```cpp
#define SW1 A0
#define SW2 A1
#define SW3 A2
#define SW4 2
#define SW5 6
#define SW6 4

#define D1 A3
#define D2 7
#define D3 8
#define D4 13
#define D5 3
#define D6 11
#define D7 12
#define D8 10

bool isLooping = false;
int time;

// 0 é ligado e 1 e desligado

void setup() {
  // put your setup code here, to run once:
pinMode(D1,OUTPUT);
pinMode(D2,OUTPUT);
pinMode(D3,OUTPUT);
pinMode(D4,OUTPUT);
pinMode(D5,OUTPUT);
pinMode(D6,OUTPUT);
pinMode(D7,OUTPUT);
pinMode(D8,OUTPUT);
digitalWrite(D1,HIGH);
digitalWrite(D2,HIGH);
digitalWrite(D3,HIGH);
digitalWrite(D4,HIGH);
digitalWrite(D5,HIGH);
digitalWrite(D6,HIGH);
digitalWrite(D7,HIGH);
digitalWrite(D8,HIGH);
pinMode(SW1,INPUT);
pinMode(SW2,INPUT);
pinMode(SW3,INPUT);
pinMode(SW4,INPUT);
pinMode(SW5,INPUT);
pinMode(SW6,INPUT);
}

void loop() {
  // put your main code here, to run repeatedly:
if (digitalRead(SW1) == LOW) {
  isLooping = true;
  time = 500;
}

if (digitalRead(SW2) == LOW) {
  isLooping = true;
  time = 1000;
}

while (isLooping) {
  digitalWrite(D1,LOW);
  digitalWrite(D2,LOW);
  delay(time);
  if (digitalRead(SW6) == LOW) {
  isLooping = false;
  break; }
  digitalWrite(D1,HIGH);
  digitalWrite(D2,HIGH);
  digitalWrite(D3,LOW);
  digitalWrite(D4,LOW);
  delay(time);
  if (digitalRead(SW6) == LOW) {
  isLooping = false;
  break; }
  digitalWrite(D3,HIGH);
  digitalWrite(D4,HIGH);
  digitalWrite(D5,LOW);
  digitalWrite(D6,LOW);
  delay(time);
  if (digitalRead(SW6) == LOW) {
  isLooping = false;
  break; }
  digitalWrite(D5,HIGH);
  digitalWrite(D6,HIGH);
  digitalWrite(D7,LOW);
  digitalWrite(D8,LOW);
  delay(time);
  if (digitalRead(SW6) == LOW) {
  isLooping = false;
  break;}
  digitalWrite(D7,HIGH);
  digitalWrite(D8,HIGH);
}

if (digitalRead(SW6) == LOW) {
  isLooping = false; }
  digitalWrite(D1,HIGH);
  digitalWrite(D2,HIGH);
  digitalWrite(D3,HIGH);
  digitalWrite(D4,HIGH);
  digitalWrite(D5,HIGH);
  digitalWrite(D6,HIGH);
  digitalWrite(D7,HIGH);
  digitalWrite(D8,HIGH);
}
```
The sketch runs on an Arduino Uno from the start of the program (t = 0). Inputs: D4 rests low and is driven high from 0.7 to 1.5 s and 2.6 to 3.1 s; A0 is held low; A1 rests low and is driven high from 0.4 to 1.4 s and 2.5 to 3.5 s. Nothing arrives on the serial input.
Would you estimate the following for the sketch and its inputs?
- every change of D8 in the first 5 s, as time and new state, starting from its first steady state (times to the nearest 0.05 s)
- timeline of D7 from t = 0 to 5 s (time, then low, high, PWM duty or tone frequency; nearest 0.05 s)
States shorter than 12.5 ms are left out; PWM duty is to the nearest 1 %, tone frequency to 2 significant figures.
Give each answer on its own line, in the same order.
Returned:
0 s high; 1 s low; 2 s high; 3 s low; 4 s high
0 s low; 1 s high; 2 s low; 3 s high; 4 s low
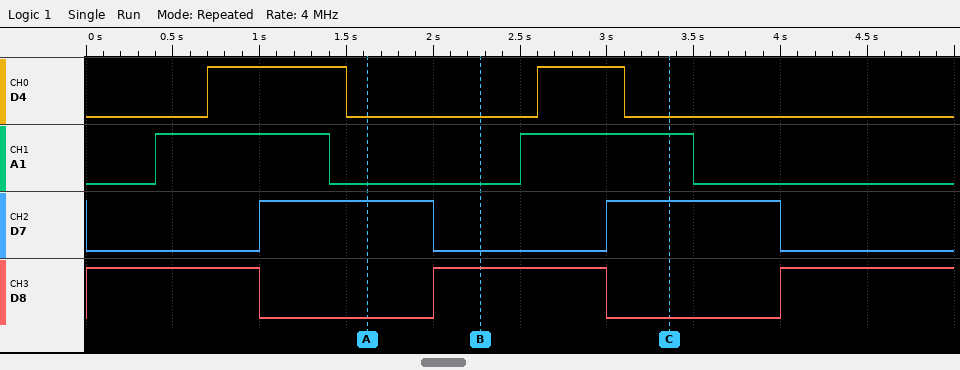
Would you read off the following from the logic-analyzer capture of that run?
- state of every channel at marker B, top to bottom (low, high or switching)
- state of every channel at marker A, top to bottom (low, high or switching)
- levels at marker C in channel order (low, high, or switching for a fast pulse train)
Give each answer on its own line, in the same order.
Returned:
D4 low, A1 low, D7 low, D8 high
D4 low, A1 low, D7 high, D8 low
D4 low, A1 high, D7 high, D8 low
